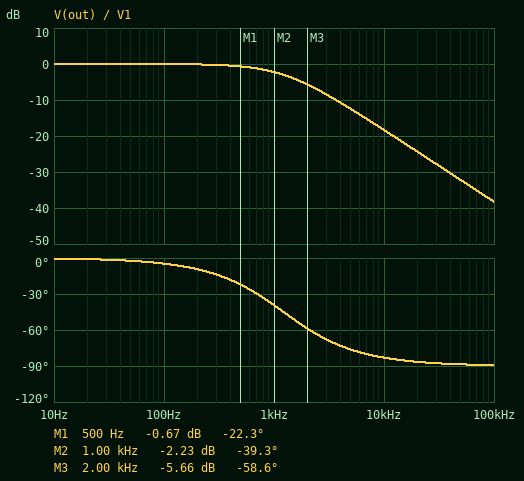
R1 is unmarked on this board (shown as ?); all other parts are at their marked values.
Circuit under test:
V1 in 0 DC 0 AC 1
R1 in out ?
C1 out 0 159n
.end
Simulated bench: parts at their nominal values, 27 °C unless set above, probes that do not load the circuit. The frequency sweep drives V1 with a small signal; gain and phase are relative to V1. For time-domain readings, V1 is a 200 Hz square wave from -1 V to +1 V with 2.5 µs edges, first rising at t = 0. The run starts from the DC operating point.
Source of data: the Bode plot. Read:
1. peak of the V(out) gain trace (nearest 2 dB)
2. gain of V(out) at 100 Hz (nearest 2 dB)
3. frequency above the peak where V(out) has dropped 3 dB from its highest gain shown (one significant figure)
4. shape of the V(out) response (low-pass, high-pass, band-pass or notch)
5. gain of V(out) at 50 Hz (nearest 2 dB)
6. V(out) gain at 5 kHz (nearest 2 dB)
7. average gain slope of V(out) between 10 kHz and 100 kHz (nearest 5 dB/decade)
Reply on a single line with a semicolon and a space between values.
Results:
0 dB; 0 dB; 1 kHz; low-pass; 0 dB; -12 dB; -20 dB/decade
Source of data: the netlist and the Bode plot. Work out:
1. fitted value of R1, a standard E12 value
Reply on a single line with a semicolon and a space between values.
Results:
820 Ω
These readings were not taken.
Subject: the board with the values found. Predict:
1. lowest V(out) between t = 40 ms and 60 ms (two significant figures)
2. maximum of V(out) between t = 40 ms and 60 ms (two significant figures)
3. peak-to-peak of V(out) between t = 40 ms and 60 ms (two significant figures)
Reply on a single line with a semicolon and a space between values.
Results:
-1.0 V; 1.0 V; 2.0 V
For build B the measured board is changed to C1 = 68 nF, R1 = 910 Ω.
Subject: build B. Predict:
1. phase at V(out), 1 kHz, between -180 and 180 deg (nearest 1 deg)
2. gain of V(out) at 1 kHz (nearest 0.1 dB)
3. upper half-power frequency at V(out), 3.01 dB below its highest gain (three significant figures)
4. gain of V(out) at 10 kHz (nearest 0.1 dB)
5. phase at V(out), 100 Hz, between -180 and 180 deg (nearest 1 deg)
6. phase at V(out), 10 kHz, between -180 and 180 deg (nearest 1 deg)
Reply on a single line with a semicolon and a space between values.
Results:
-21 deg; -0.6 dB; 2.57 kHz; -12.1 dB; -2 deg; -76 deg
